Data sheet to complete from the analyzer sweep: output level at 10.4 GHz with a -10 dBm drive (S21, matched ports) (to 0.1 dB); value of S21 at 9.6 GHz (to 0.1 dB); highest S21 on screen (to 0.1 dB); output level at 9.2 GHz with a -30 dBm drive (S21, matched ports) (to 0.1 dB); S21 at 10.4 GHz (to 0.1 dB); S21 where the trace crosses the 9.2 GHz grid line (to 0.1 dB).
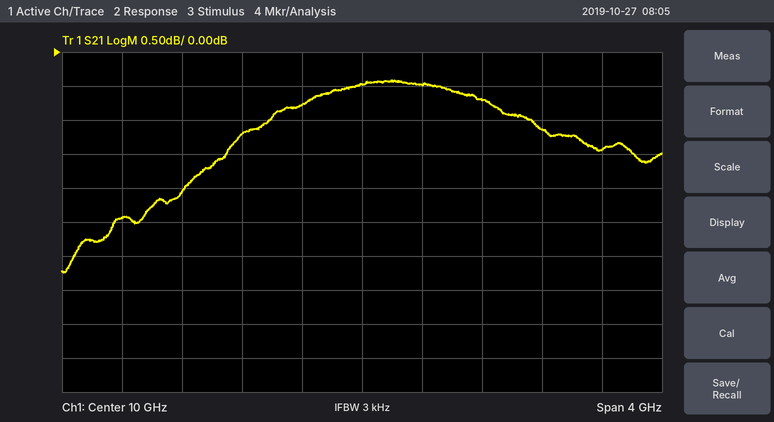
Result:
-10.5 dBm
-0.8 dB
-0.4 dB
-31.2 dBm
-0.5 dB
-1.2 dB
